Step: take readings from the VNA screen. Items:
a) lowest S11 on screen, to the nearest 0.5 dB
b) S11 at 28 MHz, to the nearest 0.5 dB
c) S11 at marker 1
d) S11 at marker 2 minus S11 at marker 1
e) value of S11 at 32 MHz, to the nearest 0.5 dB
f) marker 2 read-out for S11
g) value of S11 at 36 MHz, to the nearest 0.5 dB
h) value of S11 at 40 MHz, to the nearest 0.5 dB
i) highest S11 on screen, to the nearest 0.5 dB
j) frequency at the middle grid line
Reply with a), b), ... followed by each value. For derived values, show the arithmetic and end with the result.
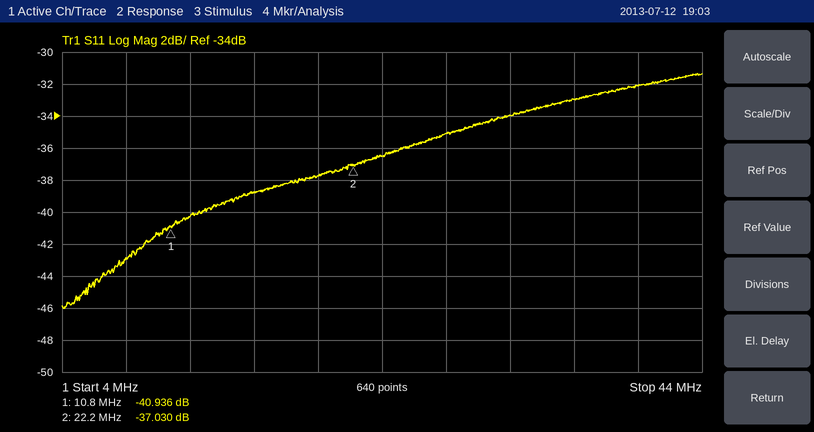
a) -46.0 dB
b) -35.0 dB
c) -40.936 dB
d) -37.03 − (-40.936) = 3.906 dB
e) -34.0 dB
f) -37.030 dB
g) -33.0 dB
h) -32.0 dB
i) -31.5 dB
j) 24 MHz
